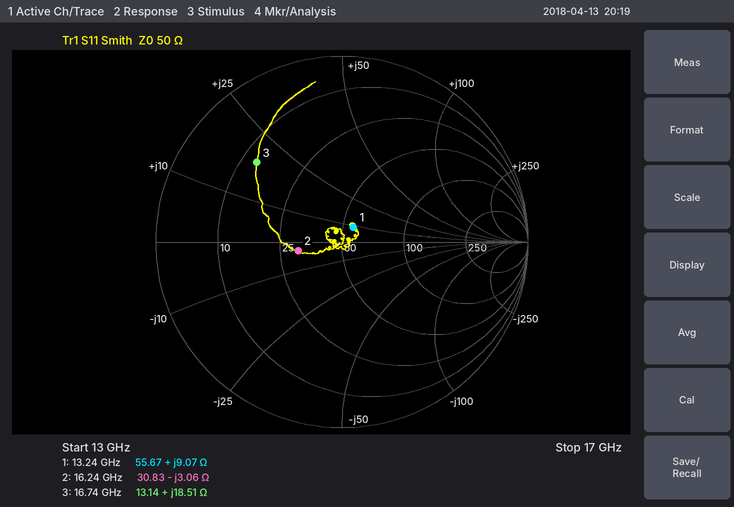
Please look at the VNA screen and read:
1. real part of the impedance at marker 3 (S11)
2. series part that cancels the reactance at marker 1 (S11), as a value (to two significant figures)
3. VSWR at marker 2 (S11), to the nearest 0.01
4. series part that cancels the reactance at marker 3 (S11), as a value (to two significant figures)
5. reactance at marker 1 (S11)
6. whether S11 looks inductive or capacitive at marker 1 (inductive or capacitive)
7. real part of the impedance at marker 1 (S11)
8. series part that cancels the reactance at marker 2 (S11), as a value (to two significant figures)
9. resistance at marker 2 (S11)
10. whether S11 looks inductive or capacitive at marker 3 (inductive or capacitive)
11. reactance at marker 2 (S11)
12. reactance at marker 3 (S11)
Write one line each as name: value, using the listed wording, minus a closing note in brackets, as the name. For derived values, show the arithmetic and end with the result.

real part of the impedance at marker 3: 13.14 Ω
series part that cancels the reactance at marker 1 (S11), as a value: C = 1/(2π × 13.24 GHz × 9.07 Ω) ≈ 1.3 pF
VSWR at marker 2 (S11), to the nearest 0.01: 1.63
series part that cancels the reactance at marker 3 (S11), as a value: C = 1/(2π × 16.74 GHz × 18.51 Ω) ≈ 514 fF, so 510 fF to two significant figures
reactance at marker 1: +9.07 Ω
whether S11 looks inductive or capacitive at marker 1: inductive
real part of the impedance at marker 1: 55.67 Ω
series part that cancels the reactance at marker 2 (S11), as a value: L = 3.06 Ω/(2π × 16.24 GHz) ≈ 30 pH
resistance at marker 2: 30.83 Ω
whether S11 looks inductive or capacitive at marker 3: inductive
reactance at marker 2: -3.06 Ω
reactance at marker 3: +18.51 Ω
